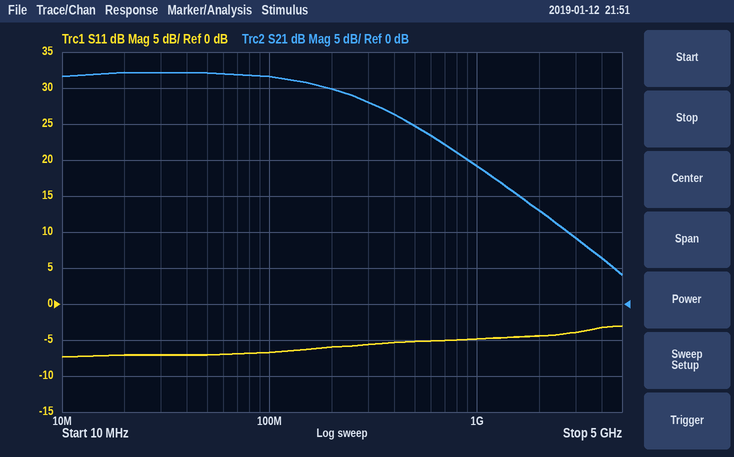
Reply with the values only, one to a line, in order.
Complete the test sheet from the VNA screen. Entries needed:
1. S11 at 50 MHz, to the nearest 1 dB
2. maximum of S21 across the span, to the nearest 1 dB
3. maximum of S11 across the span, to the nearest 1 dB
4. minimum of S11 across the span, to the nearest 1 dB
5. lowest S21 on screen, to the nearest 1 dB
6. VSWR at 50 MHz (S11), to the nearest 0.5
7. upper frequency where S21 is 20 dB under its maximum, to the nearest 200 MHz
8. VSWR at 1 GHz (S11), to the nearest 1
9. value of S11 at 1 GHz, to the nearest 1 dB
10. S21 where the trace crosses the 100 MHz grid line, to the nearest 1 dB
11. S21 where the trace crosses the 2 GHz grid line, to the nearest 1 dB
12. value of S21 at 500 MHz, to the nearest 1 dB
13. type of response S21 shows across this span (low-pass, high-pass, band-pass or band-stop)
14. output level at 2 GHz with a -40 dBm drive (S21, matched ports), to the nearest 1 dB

-7 dB
32 dB
-3 dB
-7 dB
4 dB
2.5
2.2 GHz
4
-5 dB
32 dB
13 dB
25 dB
low-pass
-27 dBm
